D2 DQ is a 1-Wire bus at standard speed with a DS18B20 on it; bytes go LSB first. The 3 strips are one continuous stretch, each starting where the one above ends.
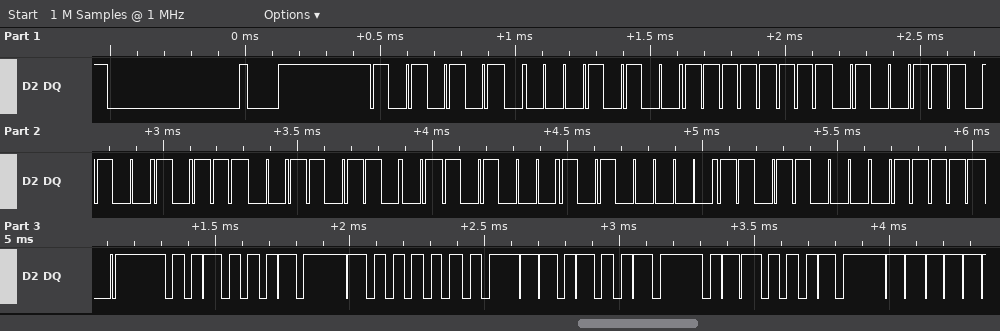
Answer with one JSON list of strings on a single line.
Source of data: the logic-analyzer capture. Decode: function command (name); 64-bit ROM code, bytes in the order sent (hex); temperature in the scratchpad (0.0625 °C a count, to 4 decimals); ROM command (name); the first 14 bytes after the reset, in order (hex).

["Read Scratchpad", "28 FF 72 E9 6C 16 05 1B", "20.2500 °C", "Match ROM", "55 28 FF 72 E9 6C 16 05 1B BE 44 01 4B 46"]
